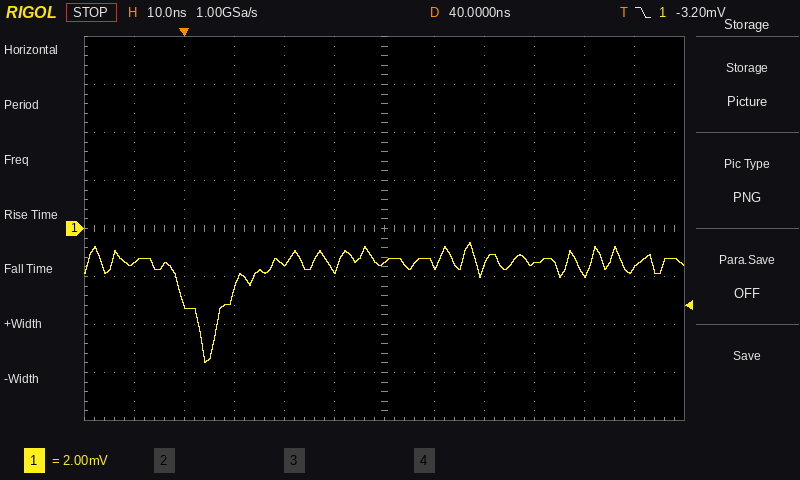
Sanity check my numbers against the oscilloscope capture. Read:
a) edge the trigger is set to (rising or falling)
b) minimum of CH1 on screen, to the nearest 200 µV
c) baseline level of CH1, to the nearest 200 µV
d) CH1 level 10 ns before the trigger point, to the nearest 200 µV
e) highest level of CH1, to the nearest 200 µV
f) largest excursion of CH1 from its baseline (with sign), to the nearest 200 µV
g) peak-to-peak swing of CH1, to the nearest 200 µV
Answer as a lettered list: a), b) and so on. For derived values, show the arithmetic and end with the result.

a) falling
b) -5.6 mV
c) -1.4 mV
d) -1.4 mV
e) -600 µV
f) -5.6 mV − (-1.4 mV) = -4.2 mV
g) -600 µV − (-5.6 mV) = 5.0 mV
